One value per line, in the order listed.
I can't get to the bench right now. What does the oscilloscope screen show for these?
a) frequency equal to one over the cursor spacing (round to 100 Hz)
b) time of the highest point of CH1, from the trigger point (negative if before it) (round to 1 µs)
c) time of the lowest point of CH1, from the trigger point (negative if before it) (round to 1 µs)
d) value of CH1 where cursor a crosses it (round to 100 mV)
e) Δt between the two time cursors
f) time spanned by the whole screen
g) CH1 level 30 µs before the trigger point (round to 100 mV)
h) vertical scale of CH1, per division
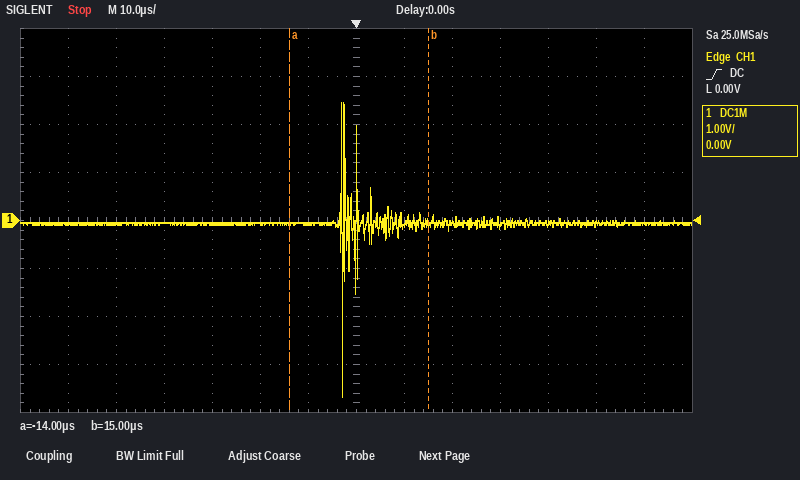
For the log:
34.5 kHz
-3 µs
-3 µs
-100 mV
29 µs
140 µs
-100 mV
1 V
